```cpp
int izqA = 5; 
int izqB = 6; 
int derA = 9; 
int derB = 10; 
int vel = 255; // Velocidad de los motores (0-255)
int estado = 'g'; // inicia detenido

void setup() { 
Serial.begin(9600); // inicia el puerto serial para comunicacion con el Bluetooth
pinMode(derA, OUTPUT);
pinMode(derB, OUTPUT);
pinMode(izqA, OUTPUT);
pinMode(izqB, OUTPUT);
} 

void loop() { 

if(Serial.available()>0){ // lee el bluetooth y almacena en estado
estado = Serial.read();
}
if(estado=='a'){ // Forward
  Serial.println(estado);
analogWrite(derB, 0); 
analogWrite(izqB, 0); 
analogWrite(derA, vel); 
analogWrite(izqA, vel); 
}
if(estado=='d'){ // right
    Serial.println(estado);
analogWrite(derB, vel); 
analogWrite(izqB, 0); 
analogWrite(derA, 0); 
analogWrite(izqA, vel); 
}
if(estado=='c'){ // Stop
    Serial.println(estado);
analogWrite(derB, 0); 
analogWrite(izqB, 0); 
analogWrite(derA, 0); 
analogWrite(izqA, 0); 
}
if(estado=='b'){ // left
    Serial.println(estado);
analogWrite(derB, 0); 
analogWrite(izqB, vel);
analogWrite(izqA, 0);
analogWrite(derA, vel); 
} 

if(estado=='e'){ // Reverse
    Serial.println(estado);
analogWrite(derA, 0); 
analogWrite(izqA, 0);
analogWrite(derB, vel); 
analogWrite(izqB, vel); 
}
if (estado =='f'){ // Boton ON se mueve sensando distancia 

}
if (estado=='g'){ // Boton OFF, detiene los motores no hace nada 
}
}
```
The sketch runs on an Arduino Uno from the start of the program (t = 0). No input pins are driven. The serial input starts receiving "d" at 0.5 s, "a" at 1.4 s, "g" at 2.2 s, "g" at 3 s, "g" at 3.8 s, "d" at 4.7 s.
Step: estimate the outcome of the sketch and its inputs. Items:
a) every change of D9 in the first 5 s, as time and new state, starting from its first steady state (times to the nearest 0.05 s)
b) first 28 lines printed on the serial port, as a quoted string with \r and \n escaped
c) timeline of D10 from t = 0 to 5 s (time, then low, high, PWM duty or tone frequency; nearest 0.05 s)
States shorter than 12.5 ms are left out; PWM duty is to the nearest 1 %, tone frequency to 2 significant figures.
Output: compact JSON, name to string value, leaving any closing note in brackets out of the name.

{"every change of D9 in the first 5 s, as time and new state, starting from its first steady state": "0 s low; 1.4 s high; 4.7 s low", "first 28 lines printed on the serial port, as a quoted string with \\r and \\n escaped": "\"100\\r\\n100\\r\\n100\\r\\n100\\r\\n100\\r\\n100\\r\\n100\\r\\n100\\r\\n100\\r\\n100\\r\\n100\\r\\n100\\r\\n100\\r\\n100\\r\\n100\\r\\n100\\r\\n100\\r\\n100\\r\\n100\\r\\n100\\r\\n100\\r\\n100\\r\\n100\\r\\n100\\r\\n100\\r\\n100\\r\\n100\\r\\n100\\r\\n\"", "timeline of D10 from t = 0 to 5 s": "0 s low; 0.5 s high; 1.4 s low; 4.7 s high"}
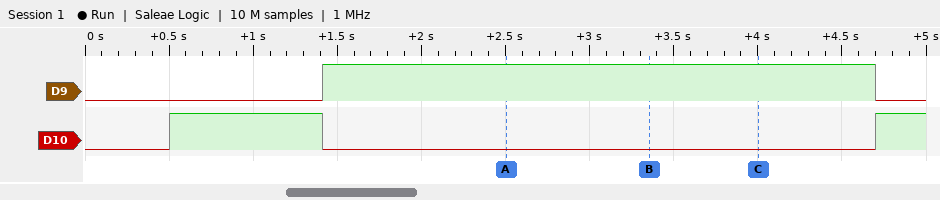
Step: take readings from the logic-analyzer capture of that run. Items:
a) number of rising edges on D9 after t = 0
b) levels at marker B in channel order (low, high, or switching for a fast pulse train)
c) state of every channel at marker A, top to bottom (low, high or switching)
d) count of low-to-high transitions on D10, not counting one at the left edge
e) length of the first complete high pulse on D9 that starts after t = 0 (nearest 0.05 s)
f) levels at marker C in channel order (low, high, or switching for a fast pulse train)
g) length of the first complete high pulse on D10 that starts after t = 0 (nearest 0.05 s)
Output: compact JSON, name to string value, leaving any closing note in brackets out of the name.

{"number of rising edges on D9 after t = 0": "1", "levels at marker B in channel order": "D9 high, D10 low", "state of every channel at marker A, top to bottom": "D9 high, D10 low", "count of low-to-high transitions on D10, not counting one at the left edge": "2", "length of the first complete high pulse on D9 that starts after t = 0": "3.30 s", "levels at marker C in channel order": "D9 high, D10 low", "length of the first complete high pulse on D10 that starts after t = 0": "0.90 s"}
